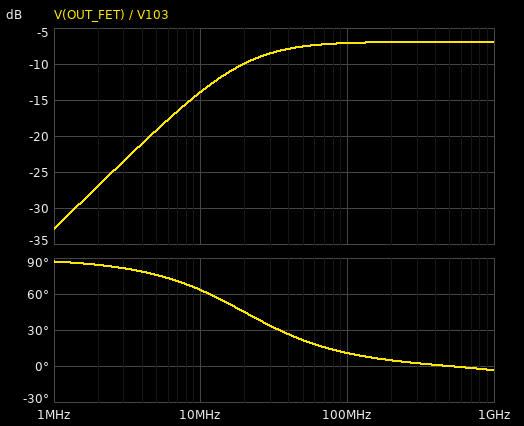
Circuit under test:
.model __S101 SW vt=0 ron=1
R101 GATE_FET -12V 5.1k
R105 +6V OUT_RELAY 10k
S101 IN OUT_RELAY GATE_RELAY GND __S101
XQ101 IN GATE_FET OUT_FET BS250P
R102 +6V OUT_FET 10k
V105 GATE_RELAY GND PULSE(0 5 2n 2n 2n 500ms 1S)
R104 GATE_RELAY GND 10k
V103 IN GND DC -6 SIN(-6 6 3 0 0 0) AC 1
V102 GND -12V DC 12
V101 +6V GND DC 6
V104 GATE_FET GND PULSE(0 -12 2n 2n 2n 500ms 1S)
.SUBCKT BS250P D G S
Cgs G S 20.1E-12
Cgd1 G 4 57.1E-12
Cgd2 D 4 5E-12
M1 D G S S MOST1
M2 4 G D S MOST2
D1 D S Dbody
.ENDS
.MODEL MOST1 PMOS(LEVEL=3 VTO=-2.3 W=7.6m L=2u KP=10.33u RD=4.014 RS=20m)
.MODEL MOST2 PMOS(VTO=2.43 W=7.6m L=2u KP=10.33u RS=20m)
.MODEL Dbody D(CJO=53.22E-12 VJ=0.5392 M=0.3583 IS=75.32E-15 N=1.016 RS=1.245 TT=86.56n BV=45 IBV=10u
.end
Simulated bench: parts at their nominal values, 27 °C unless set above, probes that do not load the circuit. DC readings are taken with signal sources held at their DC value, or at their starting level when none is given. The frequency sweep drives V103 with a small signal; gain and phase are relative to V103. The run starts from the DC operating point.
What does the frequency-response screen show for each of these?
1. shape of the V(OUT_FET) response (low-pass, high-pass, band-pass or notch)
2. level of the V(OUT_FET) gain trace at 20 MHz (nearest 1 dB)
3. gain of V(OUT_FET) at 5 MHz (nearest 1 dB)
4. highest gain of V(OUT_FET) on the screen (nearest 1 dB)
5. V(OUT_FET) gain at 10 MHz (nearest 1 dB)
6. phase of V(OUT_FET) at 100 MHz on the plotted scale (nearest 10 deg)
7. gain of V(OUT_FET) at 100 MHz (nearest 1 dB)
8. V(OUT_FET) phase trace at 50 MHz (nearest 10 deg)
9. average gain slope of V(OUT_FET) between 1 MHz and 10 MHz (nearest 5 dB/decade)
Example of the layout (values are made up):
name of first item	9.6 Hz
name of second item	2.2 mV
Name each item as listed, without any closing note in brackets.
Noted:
shape of the V(OUT_FET) response	high-pass
level of the V(OUT_FET) gain trace at 20 MHz	-10 dB
gain of V(OUT_FET) at 5 MHz	-19 dB
highest gain of V(OUT_FET) on the screen	-7 dB
V(OUT_FET) gain at 10 MHz	-14 dB
phase of V(OUT_FET) at 100 MHz on the plotted scale	10 deg
gain of V(OUT_FET) at 100 MHz	-7 dB
V(OUT_FET) phase trace at 50 MHz	20 deg
average gain slope of V(OUT_FET) between 1 MHz and 10 MHz	20 dB/decade
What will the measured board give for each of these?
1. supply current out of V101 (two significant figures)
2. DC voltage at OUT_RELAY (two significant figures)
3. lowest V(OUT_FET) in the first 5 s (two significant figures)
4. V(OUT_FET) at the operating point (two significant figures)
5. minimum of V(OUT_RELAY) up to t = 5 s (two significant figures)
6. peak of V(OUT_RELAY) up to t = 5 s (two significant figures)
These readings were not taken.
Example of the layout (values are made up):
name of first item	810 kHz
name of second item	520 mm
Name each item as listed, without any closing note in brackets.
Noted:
supply current out of V101	1.6 mA
DC voltage at OUT_RELAY	-6.0 V
lowest V(OUT_FET) in the first 5 s	-9.4 V
V(OUT_FET) at the operating point	2.4 V
minimum of V(OUT_RELAY) up to t = 5 s	-12 V
peak of V(OUT_RELAY) up to t = 5 s	6.0 V
